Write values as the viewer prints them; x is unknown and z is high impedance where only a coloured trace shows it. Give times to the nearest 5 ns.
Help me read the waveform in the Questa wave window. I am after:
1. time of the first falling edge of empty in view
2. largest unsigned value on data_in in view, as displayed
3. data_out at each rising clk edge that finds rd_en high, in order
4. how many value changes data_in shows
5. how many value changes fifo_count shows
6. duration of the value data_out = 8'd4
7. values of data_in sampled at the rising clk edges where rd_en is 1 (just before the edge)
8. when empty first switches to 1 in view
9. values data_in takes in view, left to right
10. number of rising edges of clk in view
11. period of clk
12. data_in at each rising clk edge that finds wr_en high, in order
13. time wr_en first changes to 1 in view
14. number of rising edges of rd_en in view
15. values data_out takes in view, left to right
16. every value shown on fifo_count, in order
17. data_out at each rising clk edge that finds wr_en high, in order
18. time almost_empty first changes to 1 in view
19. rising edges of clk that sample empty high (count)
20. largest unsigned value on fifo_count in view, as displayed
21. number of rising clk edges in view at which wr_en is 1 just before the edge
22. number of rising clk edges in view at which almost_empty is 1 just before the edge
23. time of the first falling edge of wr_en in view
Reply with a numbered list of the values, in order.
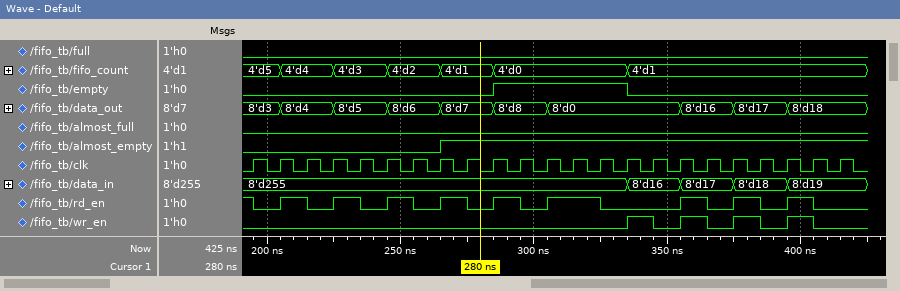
1. 335 ns
2. 8'd255
3. 8'd3, 8'd4, 8'd5, 8'd6, 8'd7, 8'd8, 8'd0, 8'd0, 8'd16, 8'd17, 8'd18
4. 4
5. 6
6. 20 ns
7. 8'd255, 8'd255, 8'd255, 8'd255, 8'd255, 8'd255, 8'd255, 8'd255, 8'd17, 8'd18, 8'd19
8. 285 ns
9. 8'd255, 8'd16, 8'd17, 8'd18, 8'd19
10. 23
11. 10 ns
12. 8'd16, 8'd17, 8'd18, 8'd19
13. 335 ns
14. 9
15. 8'd3, 8'd4, 8'd5, 8'd6, 8'd7, 8'd8, 8'd0, 8'd16, 8'd17, 8'd18
16. 4'd5, 4'd4, 4'd3, 4'd2, 4'd1, 4'd0, 4'd1
17. 8'd0, 8'd16, 8'd17, 8'd18
18. 265 ns
19. 5
20. 4'd5
21. 4
22. 15
23. 345 ns
